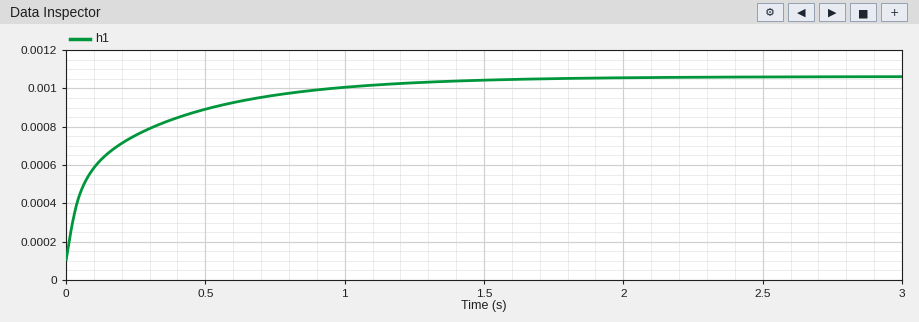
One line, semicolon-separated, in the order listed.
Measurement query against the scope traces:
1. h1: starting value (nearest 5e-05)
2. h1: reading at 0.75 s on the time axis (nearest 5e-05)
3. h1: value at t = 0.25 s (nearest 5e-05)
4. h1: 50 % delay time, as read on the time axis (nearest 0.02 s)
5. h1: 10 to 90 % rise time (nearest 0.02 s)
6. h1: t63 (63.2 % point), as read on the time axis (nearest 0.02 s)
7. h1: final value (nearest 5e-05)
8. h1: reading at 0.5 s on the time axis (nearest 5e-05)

0.00010; 0.00095; 0.00075; 0.10 s; 0.74 s; 0.20 s; 0.00105; 0.00090
